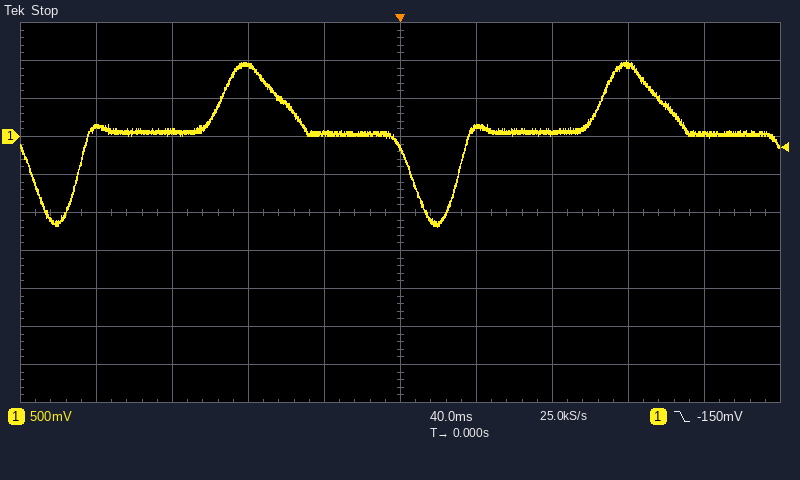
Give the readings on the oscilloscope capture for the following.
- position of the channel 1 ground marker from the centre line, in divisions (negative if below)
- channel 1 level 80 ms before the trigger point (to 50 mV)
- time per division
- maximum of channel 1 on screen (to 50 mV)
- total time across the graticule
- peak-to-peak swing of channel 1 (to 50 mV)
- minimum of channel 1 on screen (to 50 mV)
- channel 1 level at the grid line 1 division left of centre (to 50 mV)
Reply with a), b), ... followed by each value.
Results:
a) +2.0 div
b) 950 mV
c) 40 ms
d) 1.00 V
e) 400 ms
f) 2.20 V
g) -1.20 V
h) 50 mV
